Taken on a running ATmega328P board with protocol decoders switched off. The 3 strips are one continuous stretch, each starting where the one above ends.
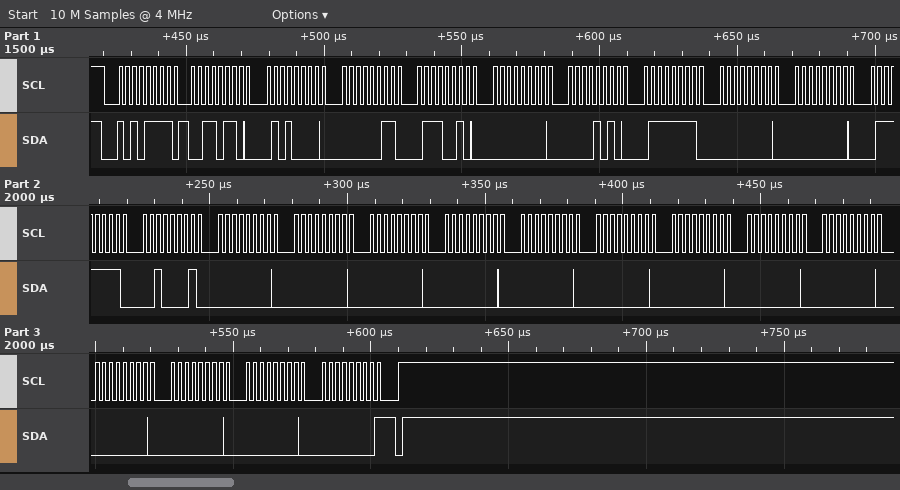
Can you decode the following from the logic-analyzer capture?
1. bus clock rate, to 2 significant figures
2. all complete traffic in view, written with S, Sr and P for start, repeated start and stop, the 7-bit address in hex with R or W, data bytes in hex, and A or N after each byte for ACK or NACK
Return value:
400 kHz
S 57R A 36 A 50 A 03 A 72 A 00 A 0A A 7F A 00 A 00 A 7F A 21 A 00 A 00 A 00 A 00 A 00 A 00 A 00 A 00 A 00 A 00 A 00 A 00 A 00 N P
